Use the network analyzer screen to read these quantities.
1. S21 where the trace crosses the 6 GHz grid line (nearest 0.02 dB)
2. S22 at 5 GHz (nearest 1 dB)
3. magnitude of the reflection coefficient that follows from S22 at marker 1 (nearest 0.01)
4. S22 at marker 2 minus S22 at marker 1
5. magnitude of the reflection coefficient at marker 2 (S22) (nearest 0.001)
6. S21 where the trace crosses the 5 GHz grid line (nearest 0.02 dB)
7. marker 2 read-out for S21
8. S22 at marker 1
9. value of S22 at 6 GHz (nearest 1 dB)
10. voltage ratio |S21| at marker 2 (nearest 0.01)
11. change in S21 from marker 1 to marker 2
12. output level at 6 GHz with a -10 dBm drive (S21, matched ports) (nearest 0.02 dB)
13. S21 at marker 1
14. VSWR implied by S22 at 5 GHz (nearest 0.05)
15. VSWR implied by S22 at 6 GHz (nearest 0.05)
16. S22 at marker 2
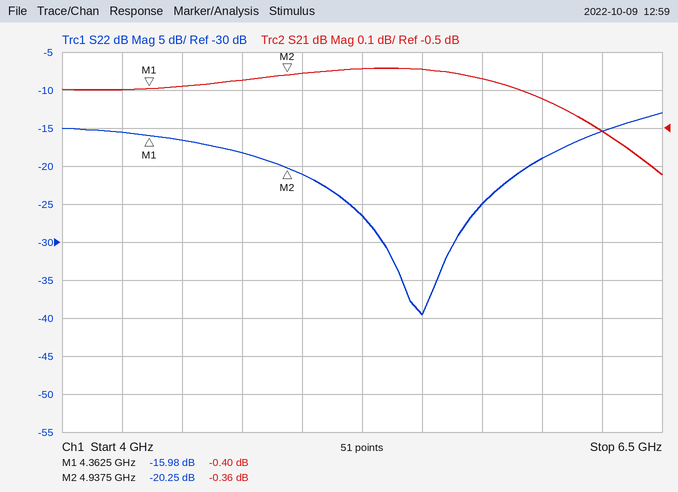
-0.42 dB
-21 dB
0.16
-4.27 dB
0.097
-0.36 dB
-0.36 dB
-15.98 dB
-19 dB
0.96
0.04 dB
-10.42 dBm
-0.40 dB
1.20
1.25
-20.25 dB
